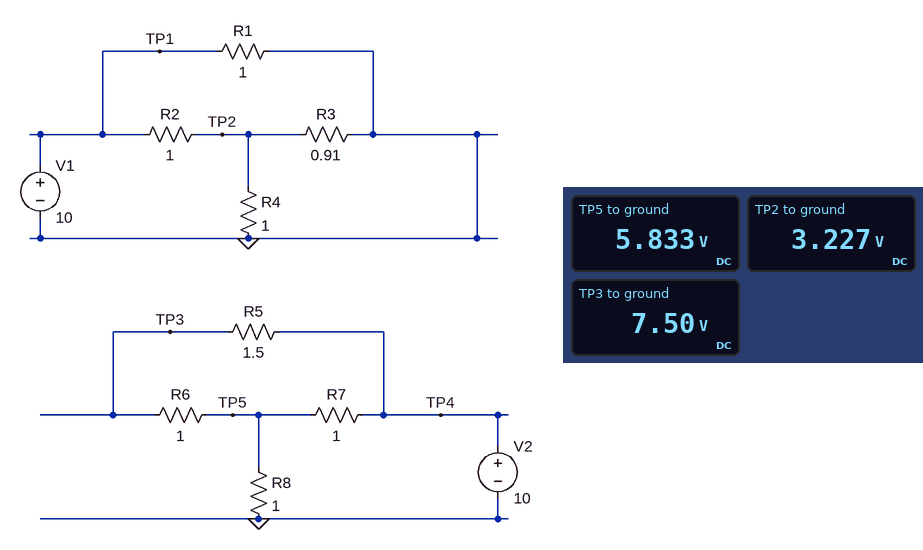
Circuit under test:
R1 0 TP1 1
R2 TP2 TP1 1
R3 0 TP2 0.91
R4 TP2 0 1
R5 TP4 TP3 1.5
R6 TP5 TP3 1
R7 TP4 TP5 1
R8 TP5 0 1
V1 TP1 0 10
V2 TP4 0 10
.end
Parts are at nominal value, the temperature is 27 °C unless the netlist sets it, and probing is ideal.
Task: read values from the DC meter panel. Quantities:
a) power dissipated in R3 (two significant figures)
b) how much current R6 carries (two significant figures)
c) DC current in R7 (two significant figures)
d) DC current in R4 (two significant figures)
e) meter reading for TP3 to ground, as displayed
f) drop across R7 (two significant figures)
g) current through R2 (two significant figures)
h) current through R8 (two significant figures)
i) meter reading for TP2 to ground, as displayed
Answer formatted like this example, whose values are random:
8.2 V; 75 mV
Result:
11 W; 1.7 A; 4.2 A; 3.2 A; 7.50 V; 4.2 V; 6.8 A; 5.8 A; 3.227 V
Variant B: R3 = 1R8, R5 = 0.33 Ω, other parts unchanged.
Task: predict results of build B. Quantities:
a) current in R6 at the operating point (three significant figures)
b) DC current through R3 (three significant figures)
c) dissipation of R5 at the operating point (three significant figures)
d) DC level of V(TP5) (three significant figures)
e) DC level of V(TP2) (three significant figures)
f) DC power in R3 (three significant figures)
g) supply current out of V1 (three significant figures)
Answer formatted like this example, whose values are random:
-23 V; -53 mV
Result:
2.73 A; 2.17 A; 2.46 W; 6.37 V; 3.91 V; 8.51 W; 16.1 A
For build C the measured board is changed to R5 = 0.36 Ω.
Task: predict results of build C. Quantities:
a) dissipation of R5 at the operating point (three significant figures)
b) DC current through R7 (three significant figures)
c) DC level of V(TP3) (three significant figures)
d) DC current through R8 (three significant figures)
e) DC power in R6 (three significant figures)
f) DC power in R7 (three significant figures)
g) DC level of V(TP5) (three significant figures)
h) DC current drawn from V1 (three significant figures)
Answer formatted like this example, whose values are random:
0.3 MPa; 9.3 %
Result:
2.60 W; 3.66 A; 9.03 V; 6.34 A; 7.23 W; 13.4 W; 6.34 V; 16.8 A
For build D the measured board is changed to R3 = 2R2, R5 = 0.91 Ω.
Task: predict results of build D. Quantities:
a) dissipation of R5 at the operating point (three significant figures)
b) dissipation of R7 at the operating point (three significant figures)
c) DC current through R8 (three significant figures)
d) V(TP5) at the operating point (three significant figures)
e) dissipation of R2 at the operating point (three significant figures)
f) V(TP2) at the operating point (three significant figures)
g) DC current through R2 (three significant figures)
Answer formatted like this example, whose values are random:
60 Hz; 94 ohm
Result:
3.92 W; 15.7 W; 6.04 A; 6.04 V; 35.1 W; 4.07 V; 5.93 A
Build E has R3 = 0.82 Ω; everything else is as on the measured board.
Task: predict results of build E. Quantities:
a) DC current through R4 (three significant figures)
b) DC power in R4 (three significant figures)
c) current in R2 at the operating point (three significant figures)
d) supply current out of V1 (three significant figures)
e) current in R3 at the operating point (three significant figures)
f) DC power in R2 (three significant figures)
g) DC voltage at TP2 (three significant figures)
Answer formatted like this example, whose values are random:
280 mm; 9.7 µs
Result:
3.11 A; 9.65 W; 6.89 A; 16.9 A; 3.79 A; 47.5 W; 3.11 V
